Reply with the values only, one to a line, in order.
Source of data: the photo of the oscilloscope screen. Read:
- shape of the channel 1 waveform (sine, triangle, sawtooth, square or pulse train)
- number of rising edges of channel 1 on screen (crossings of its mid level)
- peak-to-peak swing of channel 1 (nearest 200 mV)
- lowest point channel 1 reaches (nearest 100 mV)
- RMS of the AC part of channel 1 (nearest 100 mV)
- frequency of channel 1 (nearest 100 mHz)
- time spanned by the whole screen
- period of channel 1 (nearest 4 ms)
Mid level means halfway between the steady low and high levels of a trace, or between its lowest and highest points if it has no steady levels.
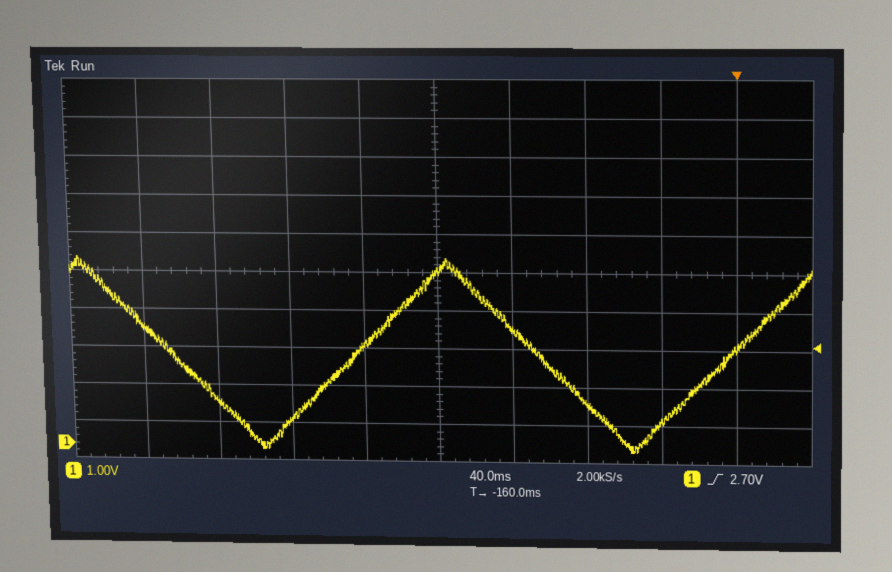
triangle
2
5.0 V
-100 mV
1.4 V
5.0 Hz
400 ms
200 ms
